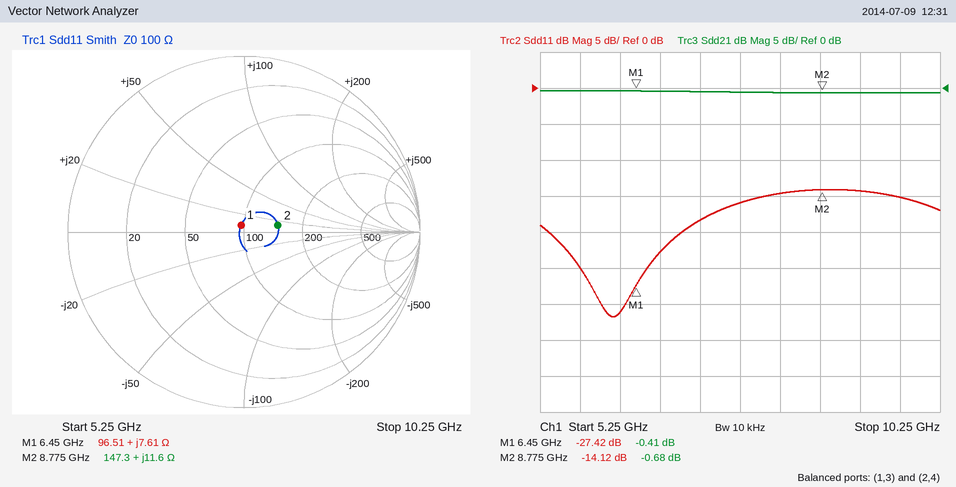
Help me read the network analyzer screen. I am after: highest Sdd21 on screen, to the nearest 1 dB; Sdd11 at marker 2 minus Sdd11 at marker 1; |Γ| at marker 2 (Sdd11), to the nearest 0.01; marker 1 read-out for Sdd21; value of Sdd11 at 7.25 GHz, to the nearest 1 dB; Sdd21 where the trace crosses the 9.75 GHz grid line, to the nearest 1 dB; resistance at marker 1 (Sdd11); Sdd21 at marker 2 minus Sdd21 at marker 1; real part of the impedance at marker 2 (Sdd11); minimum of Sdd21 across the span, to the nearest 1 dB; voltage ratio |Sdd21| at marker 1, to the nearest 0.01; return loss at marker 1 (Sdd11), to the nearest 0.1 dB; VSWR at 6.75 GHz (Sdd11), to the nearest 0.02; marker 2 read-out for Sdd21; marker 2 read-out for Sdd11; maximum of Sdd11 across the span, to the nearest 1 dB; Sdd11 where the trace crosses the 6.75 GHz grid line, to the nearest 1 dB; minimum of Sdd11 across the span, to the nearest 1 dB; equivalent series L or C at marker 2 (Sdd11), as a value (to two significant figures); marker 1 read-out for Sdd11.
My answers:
0 dB
13.30 dB
0.20
-0.41 dB
-18 dB
-1 dB
96.51 Ω
-0.27 dB
147.3 Ω
-1 dB
0.95
27.4 dB
1.16
-0.68 dB
-14.12 dB
-14 dB
-23 dB
-32 dB
210 pH
-27.42 dB
